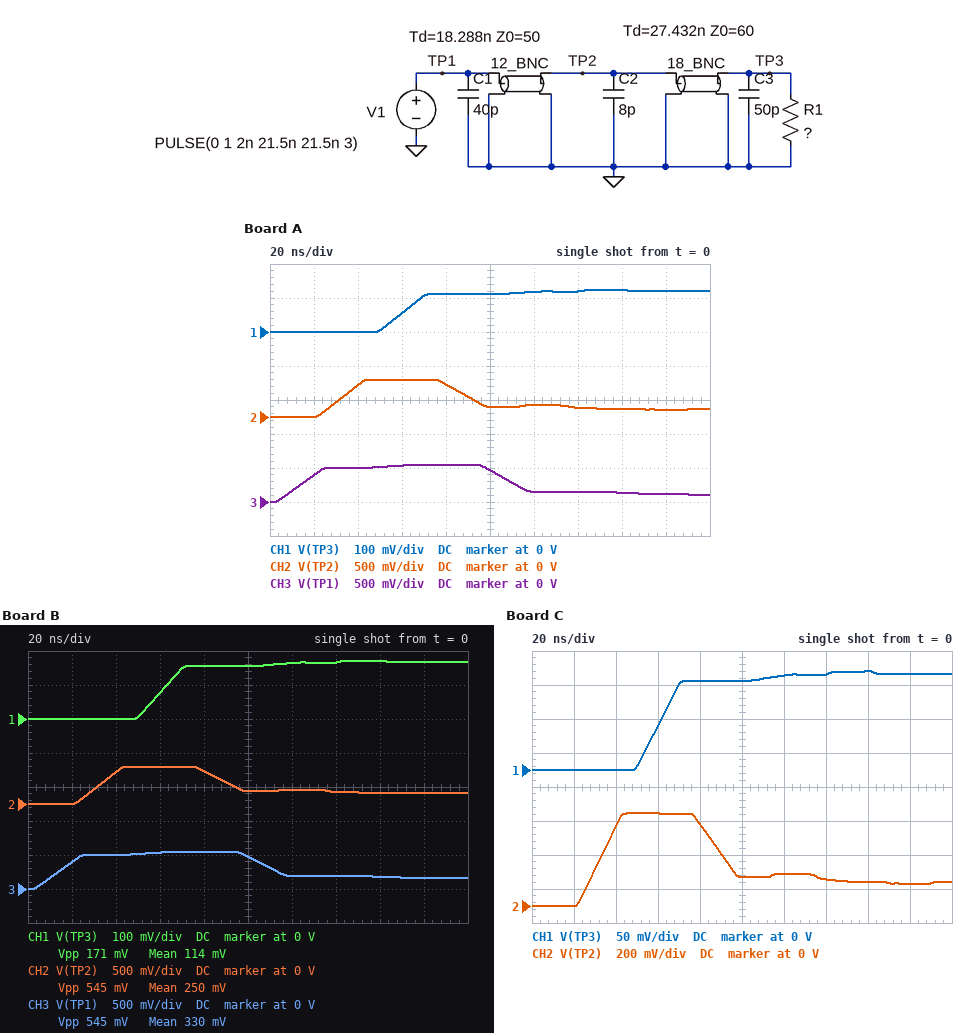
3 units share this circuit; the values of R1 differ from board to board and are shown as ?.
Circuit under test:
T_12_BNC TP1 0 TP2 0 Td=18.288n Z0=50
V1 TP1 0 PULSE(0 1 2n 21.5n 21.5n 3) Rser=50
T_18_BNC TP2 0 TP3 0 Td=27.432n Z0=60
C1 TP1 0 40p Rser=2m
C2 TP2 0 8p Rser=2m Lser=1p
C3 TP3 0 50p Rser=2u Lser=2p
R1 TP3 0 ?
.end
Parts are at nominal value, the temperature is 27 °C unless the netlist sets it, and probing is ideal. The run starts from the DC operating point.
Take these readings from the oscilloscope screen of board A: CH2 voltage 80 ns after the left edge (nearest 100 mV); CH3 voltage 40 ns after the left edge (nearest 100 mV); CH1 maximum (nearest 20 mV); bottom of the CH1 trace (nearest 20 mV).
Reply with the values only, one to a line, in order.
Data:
500 mV
500 mV
120 mV
0 V
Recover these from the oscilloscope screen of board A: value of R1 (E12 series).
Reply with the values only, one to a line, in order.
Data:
6.8 Ω
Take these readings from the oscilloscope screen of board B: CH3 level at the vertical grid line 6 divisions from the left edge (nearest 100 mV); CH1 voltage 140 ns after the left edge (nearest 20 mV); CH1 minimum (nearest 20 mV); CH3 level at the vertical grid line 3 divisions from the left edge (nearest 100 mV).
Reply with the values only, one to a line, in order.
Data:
200 mV
160 mV
0 V
500 mV
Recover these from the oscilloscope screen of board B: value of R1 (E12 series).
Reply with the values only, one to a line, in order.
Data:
10 Ω
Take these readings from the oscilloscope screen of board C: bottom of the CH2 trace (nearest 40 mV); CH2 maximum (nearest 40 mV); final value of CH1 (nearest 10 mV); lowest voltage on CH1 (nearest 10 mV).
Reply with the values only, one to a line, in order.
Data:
0 V
560 mV
140 mV
0 V
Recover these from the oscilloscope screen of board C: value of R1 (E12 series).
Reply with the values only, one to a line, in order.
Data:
8.2 Ω
